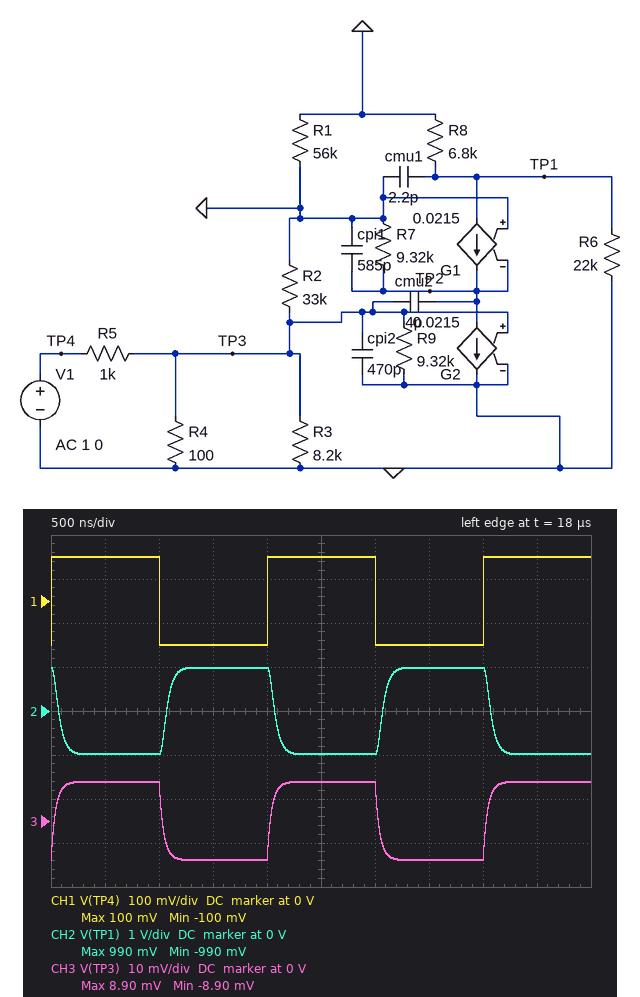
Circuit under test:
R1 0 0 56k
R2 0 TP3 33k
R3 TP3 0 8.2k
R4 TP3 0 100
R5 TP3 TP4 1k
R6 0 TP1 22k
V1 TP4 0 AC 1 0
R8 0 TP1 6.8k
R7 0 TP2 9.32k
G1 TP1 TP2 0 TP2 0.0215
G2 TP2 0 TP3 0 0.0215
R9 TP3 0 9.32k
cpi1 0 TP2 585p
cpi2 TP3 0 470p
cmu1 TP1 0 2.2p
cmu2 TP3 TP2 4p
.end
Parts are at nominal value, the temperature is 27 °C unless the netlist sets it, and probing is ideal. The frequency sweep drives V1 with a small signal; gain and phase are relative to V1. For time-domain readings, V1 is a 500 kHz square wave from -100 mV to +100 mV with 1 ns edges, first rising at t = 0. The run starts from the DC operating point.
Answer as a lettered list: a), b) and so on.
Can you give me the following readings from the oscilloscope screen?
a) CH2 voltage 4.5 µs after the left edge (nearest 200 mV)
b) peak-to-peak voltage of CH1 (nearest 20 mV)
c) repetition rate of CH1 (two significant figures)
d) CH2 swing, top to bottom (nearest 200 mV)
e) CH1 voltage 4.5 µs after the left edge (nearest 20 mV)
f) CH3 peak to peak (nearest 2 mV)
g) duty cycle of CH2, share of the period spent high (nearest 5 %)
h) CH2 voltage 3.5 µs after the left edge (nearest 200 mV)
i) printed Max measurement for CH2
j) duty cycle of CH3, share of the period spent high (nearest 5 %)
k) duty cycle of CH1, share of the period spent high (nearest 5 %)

a) -1.0 V
b) 200 mV
c) 500 kHz
d) 2.0 V
e) 100 mV
f) 18 mV
g) 50 %
h) 1.0 V
i) 990 mV
j) 50 %
k) 50 %
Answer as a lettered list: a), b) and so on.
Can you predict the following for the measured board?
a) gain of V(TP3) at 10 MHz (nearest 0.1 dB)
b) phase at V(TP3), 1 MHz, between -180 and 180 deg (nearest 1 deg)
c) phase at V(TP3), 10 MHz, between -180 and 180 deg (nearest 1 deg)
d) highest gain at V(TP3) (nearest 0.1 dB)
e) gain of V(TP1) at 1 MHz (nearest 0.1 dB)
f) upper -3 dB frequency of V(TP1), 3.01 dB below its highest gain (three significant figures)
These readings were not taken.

a) -30.1 dB
b) -15 deg
c) -69 deg
d) -21.0 dB
e) 19.4 dB
f) 2.80 MHz
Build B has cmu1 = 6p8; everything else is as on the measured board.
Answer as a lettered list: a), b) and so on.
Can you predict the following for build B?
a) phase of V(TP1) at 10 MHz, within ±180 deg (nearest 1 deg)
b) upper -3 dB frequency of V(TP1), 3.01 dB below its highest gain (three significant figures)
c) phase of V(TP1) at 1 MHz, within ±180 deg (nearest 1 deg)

a) -15 deg
b) 2.29 MHz
c) 143 deg
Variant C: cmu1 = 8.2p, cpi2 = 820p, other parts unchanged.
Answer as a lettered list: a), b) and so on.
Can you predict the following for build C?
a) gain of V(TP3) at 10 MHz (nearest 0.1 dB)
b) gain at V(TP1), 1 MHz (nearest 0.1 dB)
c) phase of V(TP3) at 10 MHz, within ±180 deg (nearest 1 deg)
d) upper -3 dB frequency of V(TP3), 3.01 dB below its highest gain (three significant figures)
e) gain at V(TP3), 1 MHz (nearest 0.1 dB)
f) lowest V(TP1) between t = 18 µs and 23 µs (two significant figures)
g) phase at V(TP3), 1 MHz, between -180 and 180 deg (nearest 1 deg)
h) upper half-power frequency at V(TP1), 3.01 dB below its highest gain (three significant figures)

a) -34.5 dB
b) 18.6 dB
c) -78 deg
d) 2.16 MHz
e) -21.9 dB
f) -990 mV
g) -25 deg
h) 1.62 MHz
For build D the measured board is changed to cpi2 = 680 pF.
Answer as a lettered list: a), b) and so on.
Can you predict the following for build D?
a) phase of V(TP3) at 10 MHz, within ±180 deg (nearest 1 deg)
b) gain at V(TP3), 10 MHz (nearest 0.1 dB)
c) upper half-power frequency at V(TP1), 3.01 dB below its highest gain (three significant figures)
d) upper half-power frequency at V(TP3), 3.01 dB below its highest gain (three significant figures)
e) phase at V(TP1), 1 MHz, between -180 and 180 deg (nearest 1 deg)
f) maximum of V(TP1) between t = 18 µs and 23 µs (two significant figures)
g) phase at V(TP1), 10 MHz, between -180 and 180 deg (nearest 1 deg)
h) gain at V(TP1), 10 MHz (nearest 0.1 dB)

a) -75 deg
b) -33.0 dB
c) 2.19 MHz
d) 2.60 MHz
e) 145 deg
f) 990 mV
g) 9 deg
h) 0.2 dB
